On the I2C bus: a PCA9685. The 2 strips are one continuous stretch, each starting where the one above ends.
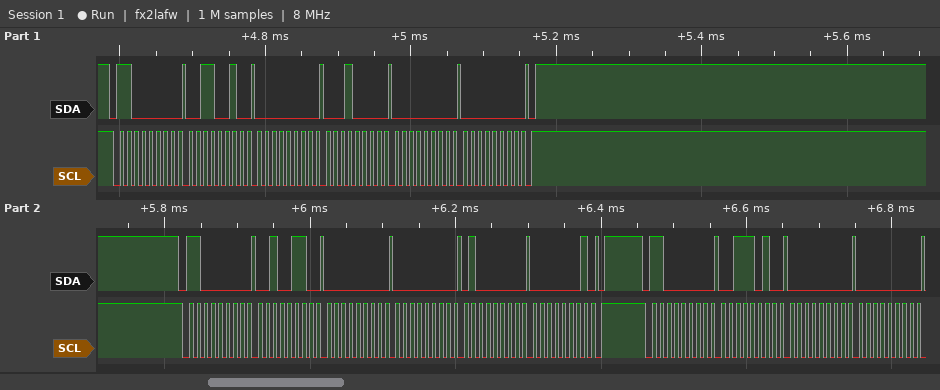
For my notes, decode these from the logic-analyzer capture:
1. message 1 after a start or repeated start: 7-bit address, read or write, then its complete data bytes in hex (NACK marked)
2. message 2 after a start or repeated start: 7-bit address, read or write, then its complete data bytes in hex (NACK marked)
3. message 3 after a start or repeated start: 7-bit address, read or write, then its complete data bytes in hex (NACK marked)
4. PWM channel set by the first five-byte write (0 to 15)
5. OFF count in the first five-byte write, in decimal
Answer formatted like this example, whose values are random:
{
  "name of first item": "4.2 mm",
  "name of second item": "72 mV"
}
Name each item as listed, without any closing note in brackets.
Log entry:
{
  "message 1 after a start or repeated start: 7-bit address, read or write, then its complete data bytes in hex": "0x60 write: 32 00 10 00 00",
  "message 2 after a start or repeated start: 7-bit address, read or write, then its complete data bytes in hex": "0x60 write: 26 00 00 40 01",
  "message 3 after a start or repeated start: 7-bit address, read or write, then its complete data bytes in hex": "0x60 write: 3A 00 00",
  "PWM channel set by the first five-byte write": "11",
  "OFF count in the first five-byte write, in decimal": "0"
}
